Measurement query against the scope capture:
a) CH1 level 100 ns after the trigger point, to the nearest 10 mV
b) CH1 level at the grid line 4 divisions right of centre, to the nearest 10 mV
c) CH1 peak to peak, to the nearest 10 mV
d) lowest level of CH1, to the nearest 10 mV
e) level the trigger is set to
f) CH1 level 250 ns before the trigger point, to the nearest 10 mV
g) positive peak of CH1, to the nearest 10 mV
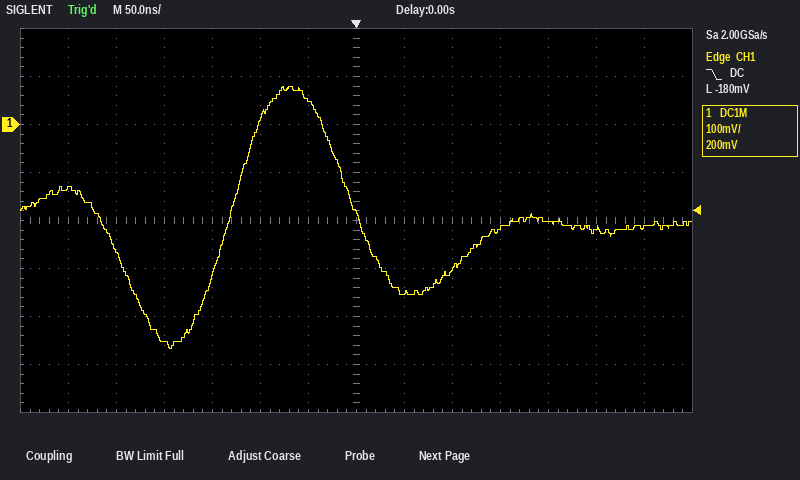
-300 mV
-200 mV
550 mV
-470 mV
-180 mV
-260 mV
80 mV
